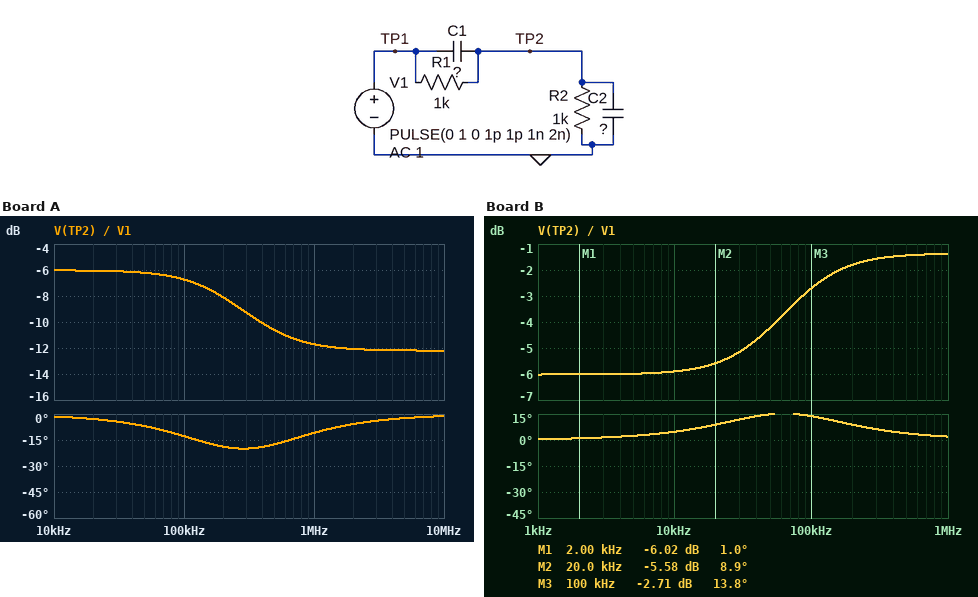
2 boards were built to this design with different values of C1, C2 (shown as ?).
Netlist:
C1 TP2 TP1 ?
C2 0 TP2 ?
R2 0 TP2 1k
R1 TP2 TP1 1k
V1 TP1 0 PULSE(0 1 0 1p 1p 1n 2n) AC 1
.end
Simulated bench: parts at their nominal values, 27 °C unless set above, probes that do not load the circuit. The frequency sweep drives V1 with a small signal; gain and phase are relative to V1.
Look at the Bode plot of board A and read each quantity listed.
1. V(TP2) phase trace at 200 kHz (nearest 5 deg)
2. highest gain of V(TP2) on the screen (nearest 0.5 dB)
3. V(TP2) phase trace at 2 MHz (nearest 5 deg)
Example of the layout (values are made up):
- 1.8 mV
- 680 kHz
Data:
- -20 deg
- -6.0 dB
- -5 deg
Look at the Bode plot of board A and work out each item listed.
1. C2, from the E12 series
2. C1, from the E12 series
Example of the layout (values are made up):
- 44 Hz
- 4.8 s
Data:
- 1.2 nF
- 390 pF
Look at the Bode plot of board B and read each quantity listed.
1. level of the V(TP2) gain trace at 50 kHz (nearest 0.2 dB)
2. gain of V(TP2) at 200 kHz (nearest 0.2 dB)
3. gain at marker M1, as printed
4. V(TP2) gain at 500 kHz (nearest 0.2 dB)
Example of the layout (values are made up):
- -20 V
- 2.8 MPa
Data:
- -4.2 dB
- -1.8 dB
- -6.02 dB
- -1.4 dB
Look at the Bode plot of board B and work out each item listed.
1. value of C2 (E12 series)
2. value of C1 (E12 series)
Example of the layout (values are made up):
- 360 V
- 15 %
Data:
- 560 pF
- 3.3 nF
